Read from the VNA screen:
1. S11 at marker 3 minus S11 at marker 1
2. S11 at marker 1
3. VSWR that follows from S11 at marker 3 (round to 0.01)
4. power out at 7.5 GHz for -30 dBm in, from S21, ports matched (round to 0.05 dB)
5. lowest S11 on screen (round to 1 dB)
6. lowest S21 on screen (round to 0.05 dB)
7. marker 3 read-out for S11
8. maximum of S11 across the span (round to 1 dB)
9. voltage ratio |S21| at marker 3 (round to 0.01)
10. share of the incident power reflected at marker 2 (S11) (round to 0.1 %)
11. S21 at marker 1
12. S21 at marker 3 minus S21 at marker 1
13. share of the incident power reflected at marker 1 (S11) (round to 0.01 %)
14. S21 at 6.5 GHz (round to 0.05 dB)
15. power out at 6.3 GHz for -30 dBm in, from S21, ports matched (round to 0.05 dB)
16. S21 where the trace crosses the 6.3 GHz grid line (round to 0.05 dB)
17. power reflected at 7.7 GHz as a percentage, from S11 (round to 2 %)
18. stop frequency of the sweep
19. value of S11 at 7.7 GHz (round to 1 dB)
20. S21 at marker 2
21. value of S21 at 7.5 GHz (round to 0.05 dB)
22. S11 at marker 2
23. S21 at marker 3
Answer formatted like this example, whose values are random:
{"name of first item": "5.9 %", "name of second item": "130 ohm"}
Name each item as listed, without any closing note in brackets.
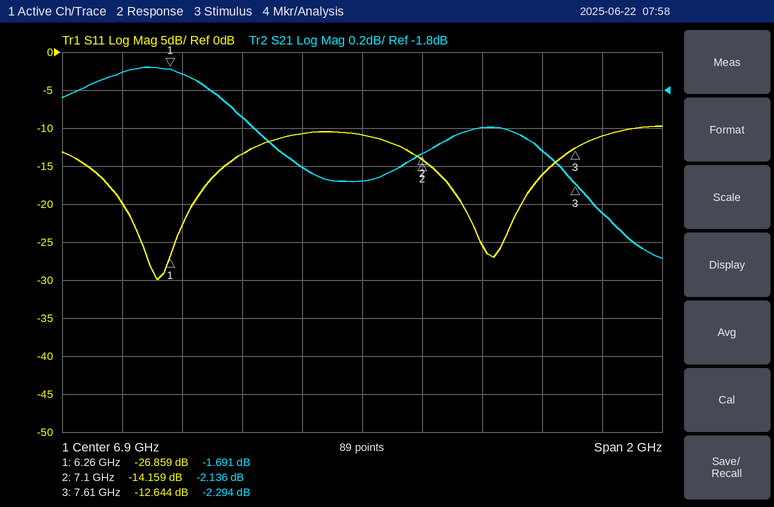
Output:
{"S11 at marker 3 minus S11 at marker 1": "14.215 dB", "S11 at marker 1": "-26.859 dB", "VSWR that follows from S11 at marker 3": "1.61", "power out at 7.5 GHz for -30 dBm in, from S21, ports matched": "-32.10 dBm", "lowest S11 on screen": "-30 dB", "lowest S21 on screen": "-2.70 dB", "marker 3 read-out for S11": "-12.644 dB", "maximum of S11 across the span": "-10 dB", "voltage ratio |S21| at marker 3": "0.77", "share of the incident power reflected at marker 2 (S11)": "3.8 %", "S21 at marker 1": "-1.691 dB", "S21 at marker 3 minus S21 at marker 1": "-0.603 dB", "share of the incident power reflected at marker 1 (S11)": "0.21 %", "S21 at 6.5 GHz": "-1.95 dB", "power out at 6.3 GHz for -30 dBm in, from S21, ports matched": "-31.70 dBm", "S21 where the trace crosses the 6.3 GHz grid line": "-1.70 dB", "power reflected at 7.7 GHz as a percentage, from S11": "8 %", "stop frequency of the sweep": "7.9 GHz", "value of S11 at 7.7 GHz": "-11 dB", "S21 at marker 2": "-2.136 dB", "value of S21 at 7.5 GHz": "-2.10 dB", "S11 at marker 2": "-14.159 dB", "S21 at marker 3": "-2.294 dB"}
